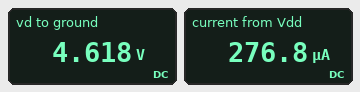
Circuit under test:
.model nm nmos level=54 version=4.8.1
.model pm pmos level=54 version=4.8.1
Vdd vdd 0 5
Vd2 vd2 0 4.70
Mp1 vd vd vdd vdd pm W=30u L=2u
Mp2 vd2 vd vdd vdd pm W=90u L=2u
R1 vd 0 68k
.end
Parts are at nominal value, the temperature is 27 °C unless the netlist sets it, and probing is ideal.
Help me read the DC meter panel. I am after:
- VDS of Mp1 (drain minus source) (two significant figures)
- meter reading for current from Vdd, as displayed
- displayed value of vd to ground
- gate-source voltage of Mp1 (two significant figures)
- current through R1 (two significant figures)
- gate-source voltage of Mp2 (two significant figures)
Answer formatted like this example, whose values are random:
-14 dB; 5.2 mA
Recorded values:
-380 mV; 276.8 µA; 4.618 V; -380 mV; 68 µA; -380 mV
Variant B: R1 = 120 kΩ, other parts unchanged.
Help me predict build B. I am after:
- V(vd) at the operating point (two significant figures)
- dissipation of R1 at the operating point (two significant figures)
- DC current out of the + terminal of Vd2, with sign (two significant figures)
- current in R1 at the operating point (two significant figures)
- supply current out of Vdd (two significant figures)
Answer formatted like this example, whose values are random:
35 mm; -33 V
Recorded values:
4.7 V; 180 µW; -120 µA; 39 µA; 160 µA
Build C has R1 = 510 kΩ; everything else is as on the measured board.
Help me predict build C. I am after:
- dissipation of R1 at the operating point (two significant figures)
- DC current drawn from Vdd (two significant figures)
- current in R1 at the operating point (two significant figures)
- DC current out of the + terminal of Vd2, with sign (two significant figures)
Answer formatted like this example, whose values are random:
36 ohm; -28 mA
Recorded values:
44 µW; 40 µA; 9.3 µA; -31 µA
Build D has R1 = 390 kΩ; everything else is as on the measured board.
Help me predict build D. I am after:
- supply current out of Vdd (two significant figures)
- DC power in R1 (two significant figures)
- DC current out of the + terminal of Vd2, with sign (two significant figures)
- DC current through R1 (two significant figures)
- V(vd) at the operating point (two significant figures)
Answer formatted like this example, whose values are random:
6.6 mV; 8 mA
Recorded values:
52 µA; 58 µW; -40 µA; 12 µA; 4.7 V
